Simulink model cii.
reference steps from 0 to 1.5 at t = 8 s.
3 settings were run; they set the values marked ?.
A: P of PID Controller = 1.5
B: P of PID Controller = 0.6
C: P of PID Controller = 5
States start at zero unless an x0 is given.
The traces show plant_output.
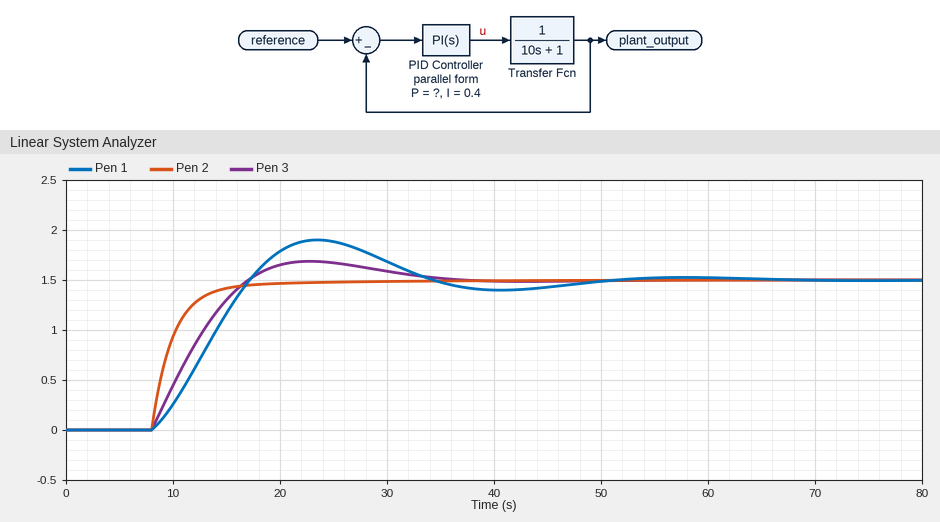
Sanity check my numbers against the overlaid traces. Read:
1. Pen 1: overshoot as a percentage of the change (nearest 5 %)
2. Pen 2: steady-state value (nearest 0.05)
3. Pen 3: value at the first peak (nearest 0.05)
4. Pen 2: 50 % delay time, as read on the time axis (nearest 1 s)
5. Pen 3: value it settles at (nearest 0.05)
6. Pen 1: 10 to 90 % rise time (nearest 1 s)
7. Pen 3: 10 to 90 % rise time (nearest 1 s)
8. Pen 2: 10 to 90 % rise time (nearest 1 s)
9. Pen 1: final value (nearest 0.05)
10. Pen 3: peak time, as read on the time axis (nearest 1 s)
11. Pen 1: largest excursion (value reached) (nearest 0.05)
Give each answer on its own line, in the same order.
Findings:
25 %
1.50
1.70
9 s
1.50
7 s
7 s
5 s
1.50
23 s
1.90
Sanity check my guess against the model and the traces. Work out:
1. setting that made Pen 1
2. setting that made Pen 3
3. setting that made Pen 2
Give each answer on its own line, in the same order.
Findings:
B
A
C
